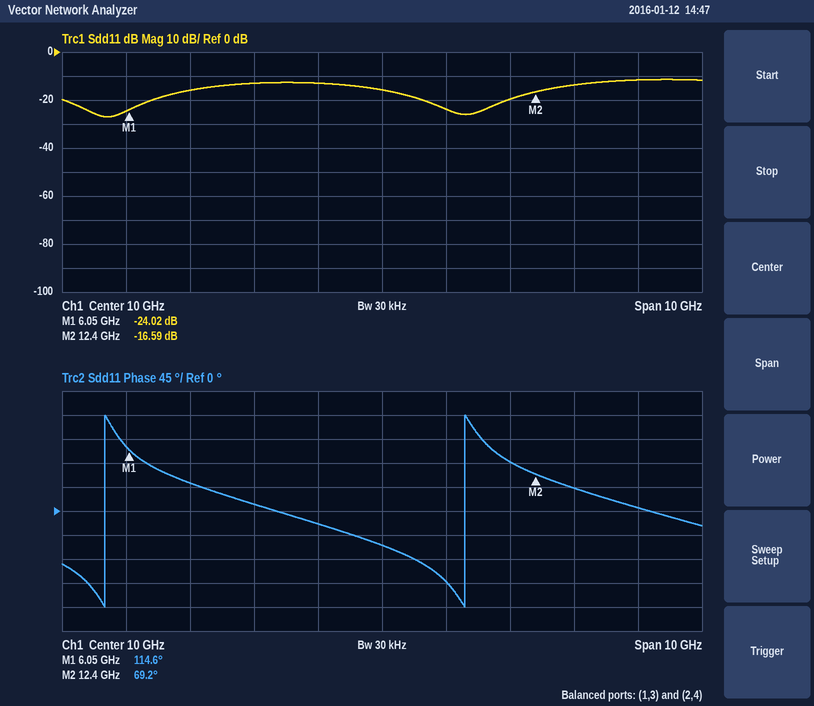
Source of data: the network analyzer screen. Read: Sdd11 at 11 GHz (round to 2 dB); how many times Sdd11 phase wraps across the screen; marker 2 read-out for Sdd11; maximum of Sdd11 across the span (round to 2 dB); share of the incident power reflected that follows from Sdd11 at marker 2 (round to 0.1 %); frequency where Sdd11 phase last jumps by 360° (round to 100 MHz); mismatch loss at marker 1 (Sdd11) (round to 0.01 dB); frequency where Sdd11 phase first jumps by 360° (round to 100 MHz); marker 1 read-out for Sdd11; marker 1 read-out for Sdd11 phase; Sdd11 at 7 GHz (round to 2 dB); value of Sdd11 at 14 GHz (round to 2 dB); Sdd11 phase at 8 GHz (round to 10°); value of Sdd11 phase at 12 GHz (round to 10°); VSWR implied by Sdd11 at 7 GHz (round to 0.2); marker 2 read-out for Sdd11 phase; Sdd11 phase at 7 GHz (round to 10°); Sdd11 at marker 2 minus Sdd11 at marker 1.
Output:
-24 dB
2
-16.59 dB
-12 dB
2.2 %
11.3 GHz
0.02 dB
5.7 GHz
-24.02 dB
114.6°
-16 dB
-12 dB
10°
90°
1.4
69.2°
50°
7.43 dB
